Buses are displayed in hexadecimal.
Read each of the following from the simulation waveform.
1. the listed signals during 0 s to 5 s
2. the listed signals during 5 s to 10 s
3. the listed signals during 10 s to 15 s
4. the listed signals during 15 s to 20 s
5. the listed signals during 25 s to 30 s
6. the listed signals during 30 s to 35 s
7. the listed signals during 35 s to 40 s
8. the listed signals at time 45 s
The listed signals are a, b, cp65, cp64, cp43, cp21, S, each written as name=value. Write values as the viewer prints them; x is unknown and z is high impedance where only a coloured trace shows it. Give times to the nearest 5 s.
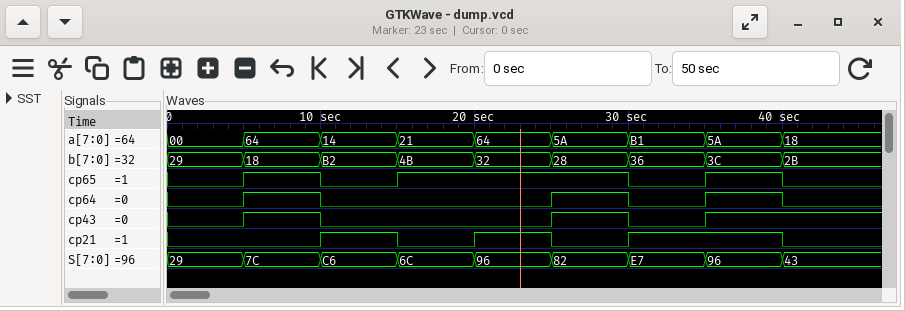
a=00, b=29, cp65=0, cp64=0, cp43=0, cp21=0, S=29
a=64, b=18, cp65=1, cp64=1, cp43=1, cp21=0, S=7C
a=14, b=B2, cp65=0, cp64=0, cp43=0, cp21=1, S=C6
a=21, b=4B, cp65=1, cp64=0, cp43=0, cp21=0, S=6C
a=5A, b=28, cp65=1, cp64=1, cp43=1, cp21=0, S=82
a=B1, b=36, cp65=0, cp64=0, cp43=0, cp21=1, S=E7
a=5A, b=3C, cp65=1, cp64=1, cp43=1, cp21=1, S=96
a=18, b=2B, cp65=0, cp64=0, cp43=1, cp21=0, S=43
